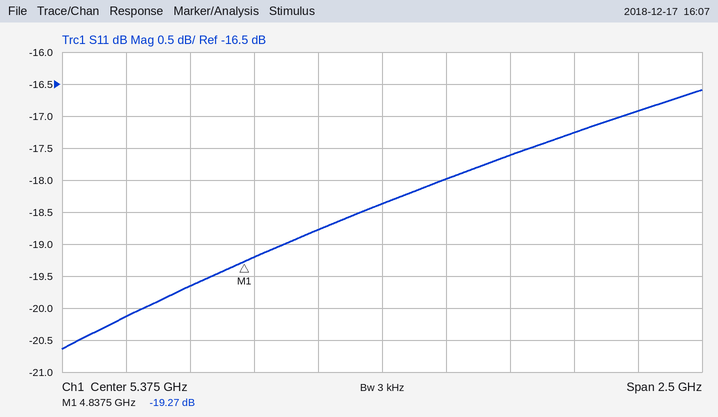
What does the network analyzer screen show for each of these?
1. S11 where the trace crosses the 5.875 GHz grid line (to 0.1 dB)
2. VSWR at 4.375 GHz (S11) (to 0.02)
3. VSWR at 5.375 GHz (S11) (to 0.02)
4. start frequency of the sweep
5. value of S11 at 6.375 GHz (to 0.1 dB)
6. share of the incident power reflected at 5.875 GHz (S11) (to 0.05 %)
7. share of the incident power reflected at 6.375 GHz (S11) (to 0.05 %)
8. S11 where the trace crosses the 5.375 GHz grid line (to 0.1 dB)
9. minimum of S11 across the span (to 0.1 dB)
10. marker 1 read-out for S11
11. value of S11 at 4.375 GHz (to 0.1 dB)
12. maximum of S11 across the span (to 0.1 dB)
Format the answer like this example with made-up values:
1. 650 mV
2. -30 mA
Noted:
1. -17.6 dB
2. 1.22
3. 1.28
4. 4.125 GHz
5. -16.9 dB
6. 1.75 %
7. 2.05 %
8. -18.4 dB
9. -20.6 dB
10. -19.27 dB
11. -20.1 dB
12. -16.6 dB
